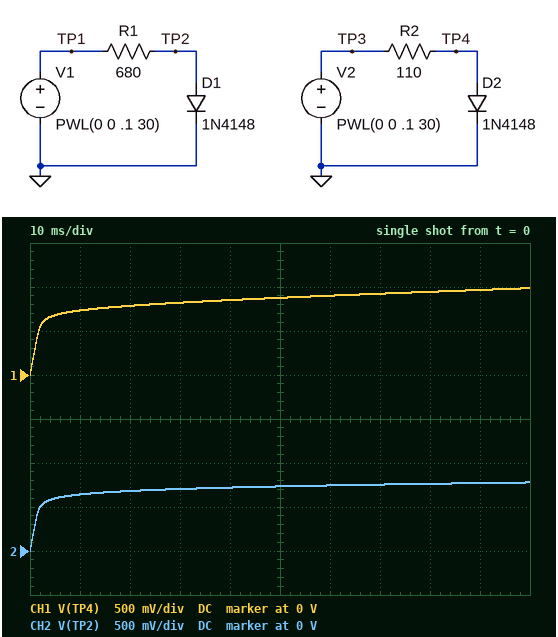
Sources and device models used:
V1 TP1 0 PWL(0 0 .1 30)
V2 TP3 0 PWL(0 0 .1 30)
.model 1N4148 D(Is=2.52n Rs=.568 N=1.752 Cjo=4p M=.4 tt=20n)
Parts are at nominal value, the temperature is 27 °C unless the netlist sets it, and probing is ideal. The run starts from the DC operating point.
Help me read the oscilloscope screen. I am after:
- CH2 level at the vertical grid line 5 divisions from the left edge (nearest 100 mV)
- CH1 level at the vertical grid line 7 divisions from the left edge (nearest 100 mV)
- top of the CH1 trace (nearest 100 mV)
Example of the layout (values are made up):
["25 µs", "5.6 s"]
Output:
["700 mV", "900 mV", "1.0 V"]
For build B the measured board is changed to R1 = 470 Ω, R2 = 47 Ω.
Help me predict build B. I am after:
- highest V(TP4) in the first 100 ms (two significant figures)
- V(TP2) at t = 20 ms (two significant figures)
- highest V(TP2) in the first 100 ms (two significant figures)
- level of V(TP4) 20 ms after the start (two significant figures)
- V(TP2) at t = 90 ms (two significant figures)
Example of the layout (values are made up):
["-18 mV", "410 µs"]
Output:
["1.2 V", "700 mV", "810 mV", "860 mV", "800 mV"]
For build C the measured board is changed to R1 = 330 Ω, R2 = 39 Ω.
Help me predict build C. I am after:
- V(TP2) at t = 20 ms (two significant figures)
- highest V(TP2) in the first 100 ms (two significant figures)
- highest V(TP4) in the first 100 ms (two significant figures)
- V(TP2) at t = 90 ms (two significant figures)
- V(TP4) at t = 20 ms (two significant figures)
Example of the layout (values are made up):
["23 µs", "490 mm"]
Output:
["720 mV", "840 mV", "1.3 V", "830 mV", "880 mV"]
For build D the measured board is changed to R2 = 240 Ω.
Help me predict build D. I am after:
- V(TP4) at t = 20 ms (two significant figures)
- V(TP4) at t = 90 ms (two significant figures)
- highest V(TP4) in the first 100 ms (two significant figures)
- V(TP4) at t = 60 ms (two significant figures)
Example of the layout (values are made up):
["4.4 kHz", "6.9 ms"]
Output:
["740 mV", "860 mV", "870 mV", "820 mV"]
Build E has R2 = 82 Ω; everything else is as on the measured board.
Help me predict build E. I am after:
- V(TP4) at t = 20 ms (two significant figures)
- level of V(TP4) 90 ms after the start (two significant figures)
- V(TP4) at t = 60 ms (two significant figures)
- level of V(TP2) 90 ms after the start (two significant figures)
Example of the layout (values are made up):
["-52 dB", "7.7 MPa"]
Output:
["810 mV", "1.0 V", "940 mV", "770 mV"]
